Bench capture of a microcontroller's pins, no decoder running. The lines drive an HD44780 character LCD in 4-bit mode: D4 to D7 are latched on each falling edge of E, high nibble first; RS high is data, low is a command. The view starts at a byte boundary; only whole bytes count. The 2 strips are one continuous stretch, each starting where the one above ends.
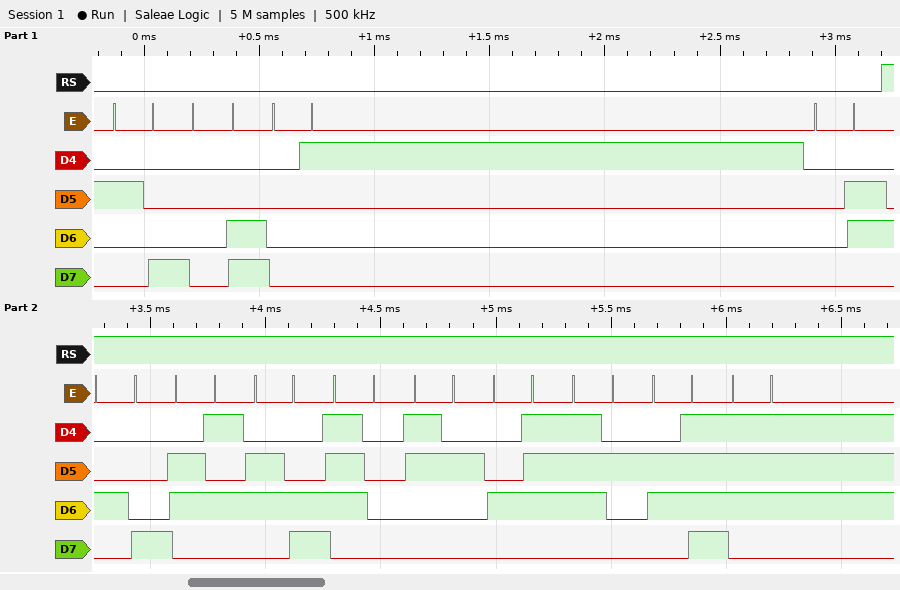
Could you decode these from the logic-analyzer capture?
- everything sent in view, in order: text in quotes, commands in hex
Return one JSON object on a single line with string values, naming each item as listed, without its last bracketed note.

{"everything sent in view, in order: text in quotes, commands in hex": "0x28 0x0C 0x01 0x06 \"Help2Grow\""}
